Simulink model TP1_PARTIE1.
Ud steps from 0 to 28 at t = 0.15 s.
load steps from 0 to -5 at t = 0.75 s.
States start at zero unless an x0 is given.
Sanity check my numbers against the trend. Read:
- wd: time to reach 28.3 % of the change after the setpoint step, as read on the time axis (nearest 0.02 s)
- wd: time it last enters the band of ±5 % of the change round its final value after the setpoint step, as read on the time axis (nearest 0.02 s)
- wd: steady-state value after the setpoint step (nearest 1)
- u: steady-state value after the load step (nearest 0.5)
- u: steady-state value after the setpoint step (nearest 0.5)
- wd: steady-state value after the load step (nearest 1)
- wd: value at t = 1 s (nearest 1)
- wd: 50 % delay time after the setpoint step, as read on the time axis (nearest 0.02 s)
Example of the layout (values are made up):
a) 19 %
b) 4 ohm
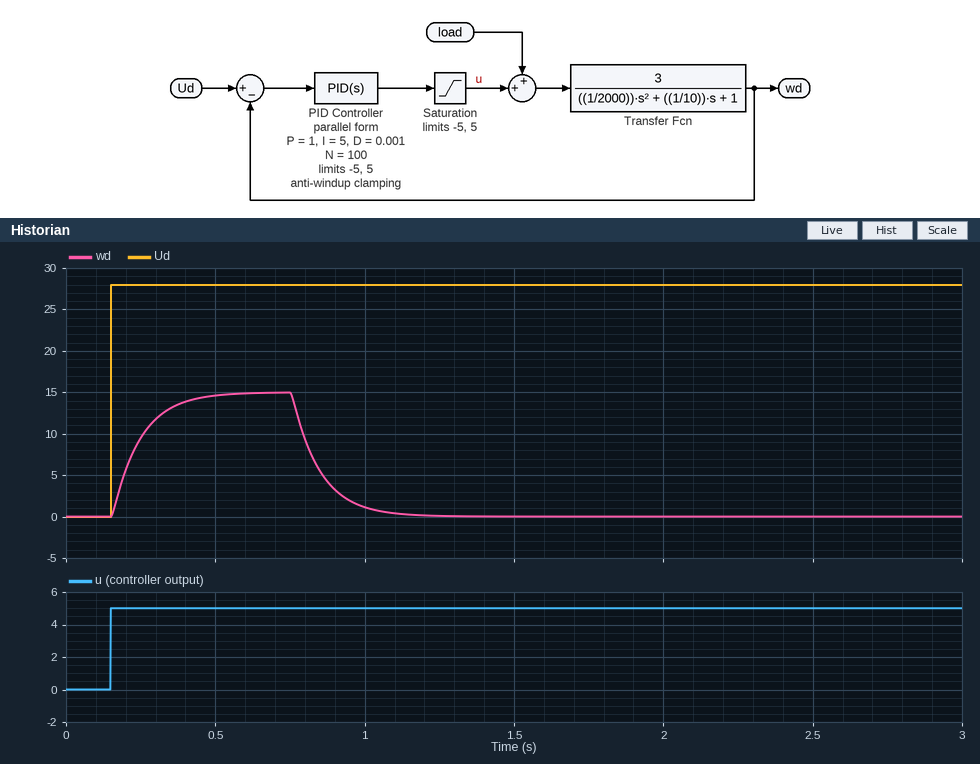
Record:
a) 0.18 s
b) 0.44 s
c) 15
d) 5.0
e) 5.0
f) 0
g) 1
h) 0.22 s
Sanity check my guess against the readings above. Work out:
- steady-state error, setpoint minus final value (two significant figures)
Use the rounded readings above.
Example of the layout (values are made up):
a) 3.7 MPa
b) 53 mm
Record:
a) 13
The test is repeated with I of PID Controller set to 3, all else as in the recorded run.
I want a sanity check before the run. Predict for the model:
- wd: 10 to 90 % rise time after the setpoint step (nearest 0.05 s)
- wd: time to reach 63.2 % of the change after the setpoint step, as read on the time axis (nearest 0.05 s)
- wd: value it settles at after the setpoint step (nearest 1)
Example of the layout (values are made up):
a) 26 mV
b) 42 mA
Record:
a) 0.20 s
b) 0.25 s
c) 15
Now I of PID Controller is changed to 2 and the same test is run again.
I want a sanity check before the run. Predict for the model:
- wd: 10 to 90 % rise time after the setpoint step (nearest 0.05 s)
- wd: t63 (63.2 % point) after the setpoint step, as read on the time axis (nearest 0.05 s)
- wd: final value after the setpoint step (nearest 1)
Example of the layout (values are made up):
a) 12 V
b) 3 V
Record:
a) 0.20 s
b) 0.25 s
c) 15
